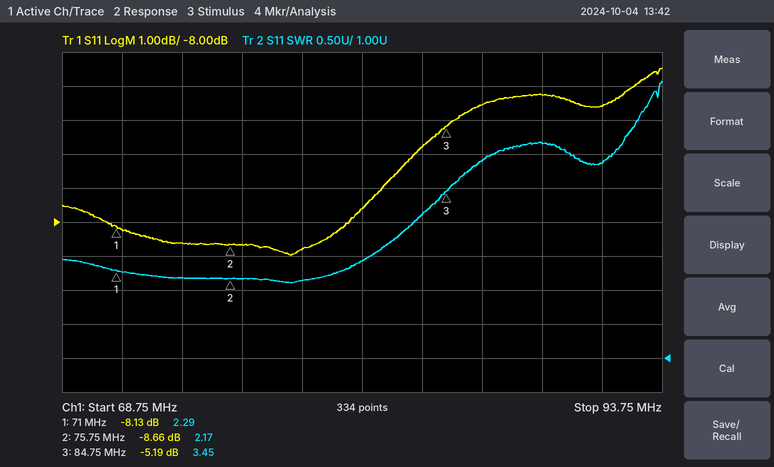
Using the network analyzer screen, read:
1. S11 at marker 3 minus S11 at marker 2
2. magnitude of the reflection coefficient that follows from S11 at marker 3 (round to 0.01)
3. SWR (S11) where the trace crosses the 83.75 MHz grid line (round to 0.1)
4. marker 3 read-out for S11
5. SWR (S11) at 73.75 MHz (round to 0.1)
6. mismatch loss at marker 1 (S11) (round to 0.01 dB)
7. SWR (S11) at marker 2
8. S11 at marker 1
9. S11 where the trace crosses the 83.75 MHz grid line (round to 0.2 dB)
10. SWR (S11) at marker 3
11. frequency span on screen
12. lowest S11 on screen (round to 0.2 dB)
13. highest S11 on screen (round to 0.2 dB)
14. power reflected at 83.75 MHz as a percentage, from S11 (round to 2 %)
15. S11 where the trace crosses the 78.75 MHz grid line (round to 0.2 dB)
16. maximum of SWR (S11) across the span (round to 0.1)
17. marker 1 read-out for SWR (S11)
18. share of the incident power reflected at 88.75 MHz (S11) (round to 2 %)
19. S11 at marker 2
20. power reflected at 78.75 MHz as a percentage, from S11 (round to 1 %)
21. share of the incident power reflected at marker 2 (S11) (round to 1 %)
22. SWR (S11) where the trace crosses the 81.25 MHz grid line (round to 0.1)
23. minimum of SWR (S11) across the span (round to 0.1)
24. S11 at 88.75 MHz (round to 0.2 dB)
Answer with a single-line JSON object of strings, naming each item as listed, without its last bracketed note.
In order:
{"S11 at marker 3 minus S11 at marker 2": "3.47 dB", "magnitude of the reflection coefficient that follows from S11 at marker 3": "0.55", "SWR (S11) where the trace crosses the 83.75 MHz grid line": "3.1", "marker 3 read-out for S11": "-5.19 dB", "SWR (S11) at 73.75 MHz": "2.2", "mismatch loss at marker 1 (S11)": "0.73 dB", "SWR (S11) at marker 2": "2.17", "S11 at marker 1": "-8.13 dB", "S11 where the trace crosses the 83.75 MHz grid line": "-5.8 dB", "SWR (S11) at marker 3": "3.45", "frequency span on screen": "25 MHz", "lowest S11 on screen": "-9.0 dB", "highest S11 on screen": "-3.4 dB", "power reflected at 83.75 MHz as a percentage, from S11": "26 %", "S11 where the trace crosses the 78.75 MHz grid line": "-8.8 dB", "maximum of SWR (S11) across the span": "5.1", "marker 1 read-out for SWR": "2.29", "share of the incident power reflected at 88.75 MHz (S11)": "38 %", "S11 at marker 2": "-8.66 dB", "power reflected at 78.75 MHz as a percentage, from S11": "13 %", "share of the incident power reflected at marker 2 (S11)": "14 %", "SWR (S11) where the trace crosses the 81.25 MHz grid line": "2.4", "minimum of SWR (S11) across the span": "2.1", "S11 at 88.75 MHz": "-4.2 dB"}
